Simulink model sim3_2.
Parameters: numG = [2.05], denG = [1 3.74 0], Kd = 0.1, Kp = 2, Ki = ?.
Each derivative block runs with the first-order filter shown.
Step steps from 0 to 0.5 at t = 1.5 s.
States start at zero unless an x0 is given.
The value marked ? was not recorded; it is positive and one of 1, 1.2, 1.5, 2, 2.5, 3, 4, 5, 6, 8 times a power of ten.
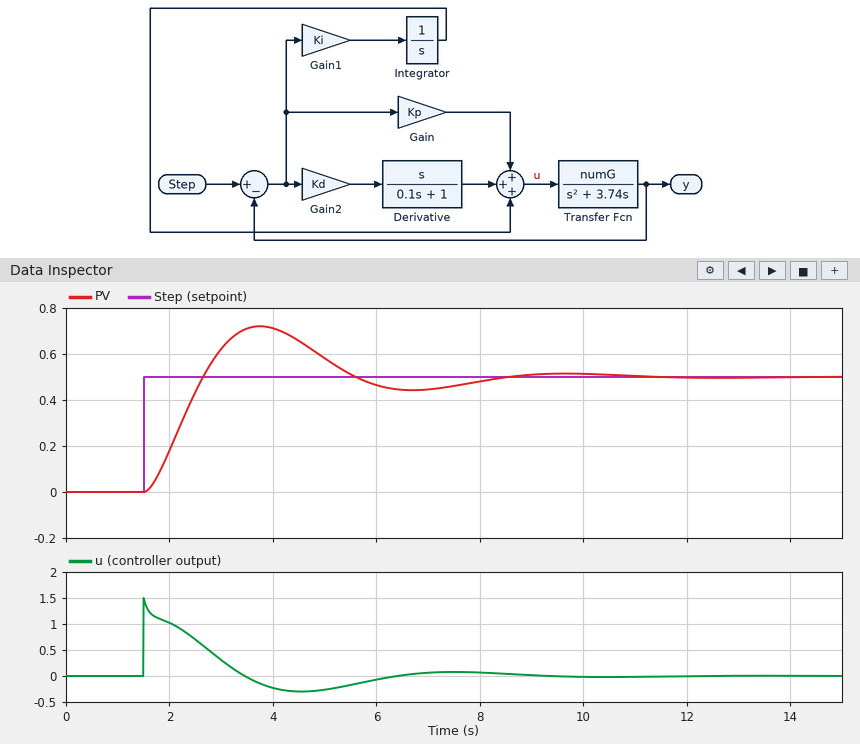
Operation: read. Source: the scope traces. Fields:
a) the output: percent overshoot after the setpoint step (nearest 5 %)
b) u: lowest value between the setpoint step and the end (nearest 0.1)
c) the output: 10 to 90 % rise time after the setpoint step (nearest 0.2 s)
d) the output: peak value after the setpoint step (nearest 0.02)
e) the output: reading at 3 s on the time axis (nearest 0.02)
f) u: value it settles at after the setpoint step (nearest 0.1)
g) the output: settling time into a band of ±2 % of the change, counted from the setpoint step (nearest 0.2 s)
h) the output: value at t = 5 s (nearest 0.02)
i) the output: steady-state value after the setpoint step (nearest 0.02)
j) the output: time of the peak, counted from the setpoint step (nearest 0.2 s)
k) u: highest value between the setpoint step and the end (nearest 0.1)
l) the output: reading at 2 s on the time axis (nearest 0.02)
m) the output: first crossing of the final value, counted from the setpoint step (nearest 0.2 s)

45 %
-0.3
0.8 s
0.72
0.62
0.0
9.0 s
0.58
0.50
2.2 s
1.5
0.18
1.2 s
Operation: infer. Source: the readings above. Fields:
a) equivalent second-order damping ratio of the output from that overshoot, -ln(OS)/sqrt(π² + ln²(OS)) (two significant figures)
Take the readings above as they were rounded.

0.25
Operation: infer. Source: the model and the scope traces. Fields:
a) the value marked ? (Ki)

2
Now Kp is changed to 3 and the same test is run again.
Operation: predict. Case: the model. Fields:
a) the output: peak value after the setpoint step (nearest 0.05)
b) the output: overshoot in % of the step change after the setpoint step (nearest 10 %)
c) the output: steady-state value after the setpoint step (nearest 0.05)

0.65
30 %
0.50
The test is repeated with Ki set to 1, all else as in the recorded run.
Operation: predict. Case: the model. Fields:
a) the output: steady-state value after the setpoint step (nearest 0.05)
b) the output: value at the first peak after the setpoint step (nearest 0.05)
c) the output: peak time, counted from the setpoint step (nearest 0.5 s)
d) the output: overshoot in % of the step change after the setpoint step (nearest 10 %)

0.50
0.65
2.5 s
30 %
